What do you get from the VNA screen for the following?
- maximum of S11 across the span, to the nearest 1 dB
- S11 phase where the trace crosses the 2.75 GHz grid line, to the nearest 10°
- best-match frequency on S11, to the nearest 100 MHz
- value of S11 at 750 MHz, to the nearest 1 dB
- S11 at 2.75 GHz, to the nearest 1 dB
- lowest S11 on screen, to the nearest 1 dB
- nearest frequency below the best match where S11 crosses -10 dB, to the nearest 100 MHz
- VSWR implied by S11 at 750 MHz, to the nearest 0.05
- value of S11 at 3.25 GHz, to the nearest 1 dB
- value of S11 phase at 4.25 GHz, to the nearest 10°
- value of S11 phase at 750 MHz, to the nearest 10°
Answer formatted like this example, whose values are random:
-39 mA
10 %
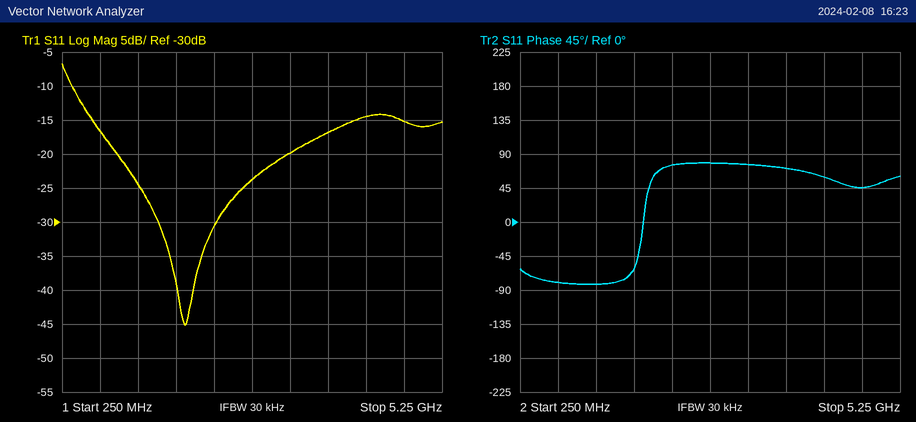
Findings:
-7 dB
80°
1.9 GHz
-17 dB
-24 dB
-45 dB
400 MHz
1.35
-20 dB
60°
-80°
